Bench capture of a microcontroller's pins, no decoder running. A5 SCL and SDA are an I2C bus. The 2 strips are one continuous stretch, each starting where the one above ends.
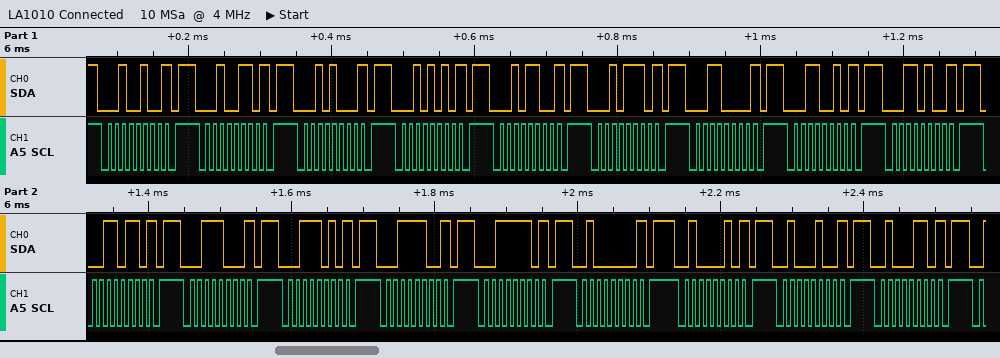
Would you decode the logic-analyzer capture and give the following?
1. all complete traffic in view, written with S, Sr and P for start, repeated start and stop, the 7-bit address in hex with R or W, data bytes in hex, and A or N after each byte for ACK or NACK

S 12W N P S 13W N P S 14W N P S 15W N P S 16W N P S 17W N P S 18W N P S 19W N P S 1AW N P S 1BW N P S 1CW N P S 1DW N P S 1EW N P S 1FW N P S 20W N P S 21W N P S 22W N P S 23W N P
